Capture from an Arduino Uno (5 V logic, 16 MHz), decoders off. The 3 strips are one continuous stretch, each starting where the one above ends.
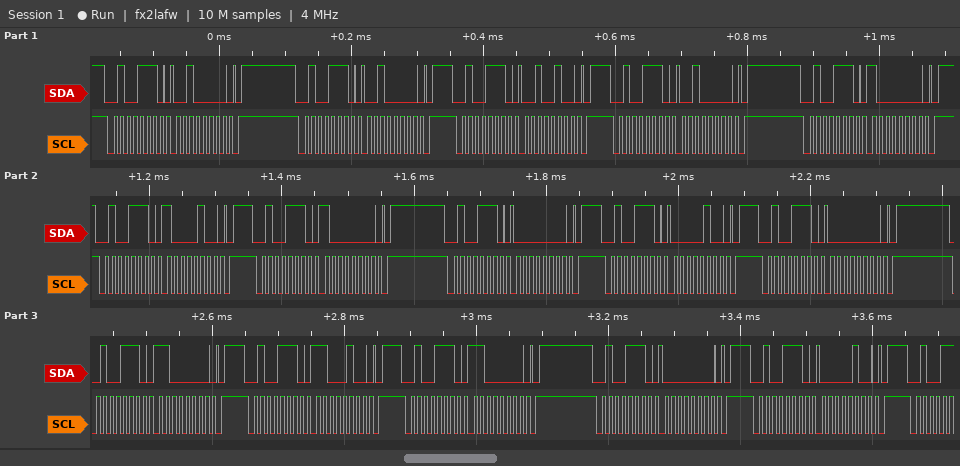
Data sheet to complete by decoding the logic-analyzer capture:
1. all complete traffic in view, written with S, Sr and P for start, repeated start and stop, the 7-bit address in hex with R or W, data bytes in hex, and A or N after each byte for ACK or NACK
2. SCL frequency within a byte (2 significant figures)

S 27W A 20 A P S 27W A 20 A P S 27W A 24 A P S 27W A 20 A P S 27W A 80 A P S 27W A 84 A P S 27W A 80 A P S 27W A 00 A P S 27W A 04 A P S 27W A 00 A P S 27W A C0 A P S 27W A C4 A P S 27W A C0 A P S 27W A 00 A P S 27W A 04 A P
100 kHz
